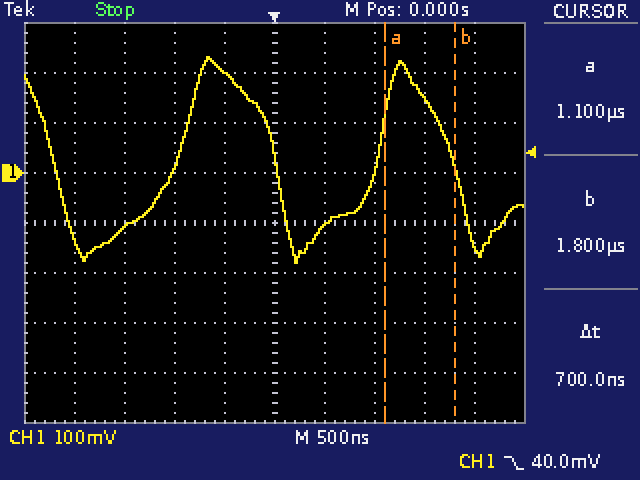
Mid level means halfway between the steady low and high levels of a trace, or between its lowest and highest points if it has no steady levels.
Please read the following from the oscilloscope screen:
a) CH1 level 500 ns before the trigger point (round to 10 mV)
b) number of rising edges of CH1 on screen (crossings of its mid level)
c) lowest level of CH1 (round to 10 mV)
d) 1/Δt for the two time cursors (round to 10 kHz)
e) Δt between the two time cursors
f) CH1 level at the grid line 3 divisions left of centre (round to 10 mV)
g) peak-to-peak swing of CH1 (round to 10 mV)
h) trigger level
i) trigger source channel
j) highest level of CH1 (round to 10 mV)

200 mV
2
-180 mV
1.43 MHz
700 ns
-110 mV
410 mV
40.0 mV
CH1
230 mV
